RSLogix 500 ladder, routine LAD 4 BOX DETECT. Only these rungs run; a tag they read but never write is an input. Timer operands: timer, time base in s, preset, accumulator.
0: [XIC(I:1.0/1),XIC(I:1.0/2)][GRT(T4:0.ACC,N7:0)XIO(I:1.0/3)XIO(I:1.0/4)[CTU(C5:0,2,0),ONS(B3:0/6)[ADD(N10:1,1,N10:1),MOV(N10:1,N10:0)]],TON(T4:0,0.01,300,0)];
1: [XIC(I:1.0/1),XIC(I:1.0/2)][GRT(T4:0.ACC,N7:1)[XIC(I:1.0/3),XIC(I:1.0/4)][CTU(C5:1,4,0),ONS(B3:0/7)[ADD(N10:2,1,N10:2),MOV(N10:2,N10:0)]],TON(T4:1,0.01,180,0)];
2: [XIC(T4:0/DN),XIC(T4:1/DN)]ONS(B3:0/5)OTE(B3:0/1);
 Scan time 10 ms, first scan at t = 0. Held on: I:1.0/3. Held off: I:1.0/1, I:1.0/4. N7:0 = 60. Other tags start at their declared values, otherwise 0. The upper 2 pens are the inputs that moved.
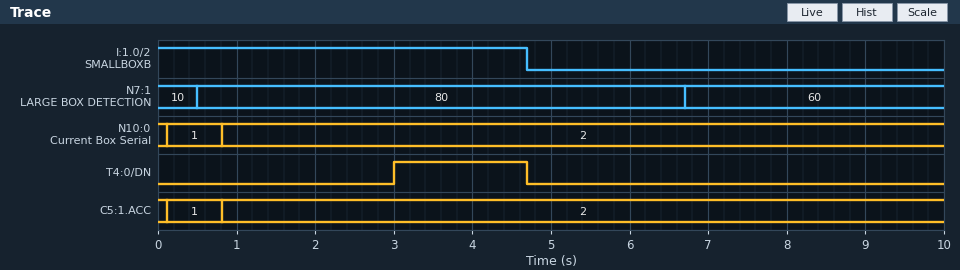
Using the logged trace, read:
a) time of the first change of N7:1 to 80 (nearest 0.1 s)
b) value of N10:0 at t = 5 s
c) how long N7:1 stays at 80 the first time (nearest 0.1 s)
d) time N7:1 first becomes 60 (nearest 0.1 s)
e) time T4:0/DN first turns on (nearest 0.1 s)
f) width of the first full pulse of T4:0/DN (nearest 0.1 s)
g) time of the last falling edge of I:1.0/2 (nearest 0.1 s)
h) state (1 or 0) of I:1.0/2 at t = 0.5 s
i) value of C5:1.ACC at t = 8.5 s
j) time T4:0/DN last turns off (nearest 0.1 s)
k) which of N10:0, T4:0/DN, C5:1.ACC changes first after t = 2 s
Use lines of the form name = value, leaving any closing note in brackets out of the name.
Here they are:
time of the first change of N7:1 to 80 = 0.5 s
value of N10:0 at t = 5 s = 2
how long N7:1 stays at 80 the first time = 6.2 s
time N7:1 first becomes 60 = 6.7 s
time T4:0/DN first turns on = 3.0 s
width of the first full pulse of T4:0/DN = 1.7 s
time of the last falling edge of I:1.0/2 = 4.7 s
state (1 or 0) of I:1.0/2 at t = 0.5 s = 1
value of C5:1.ACC at t = 8.5 s = 2
time T4:0/DN last turns off = 4.7 s
which of N10:0, T4:0/DN, C5:1.ACC changes first after t = 2 s = T4:0/DN
